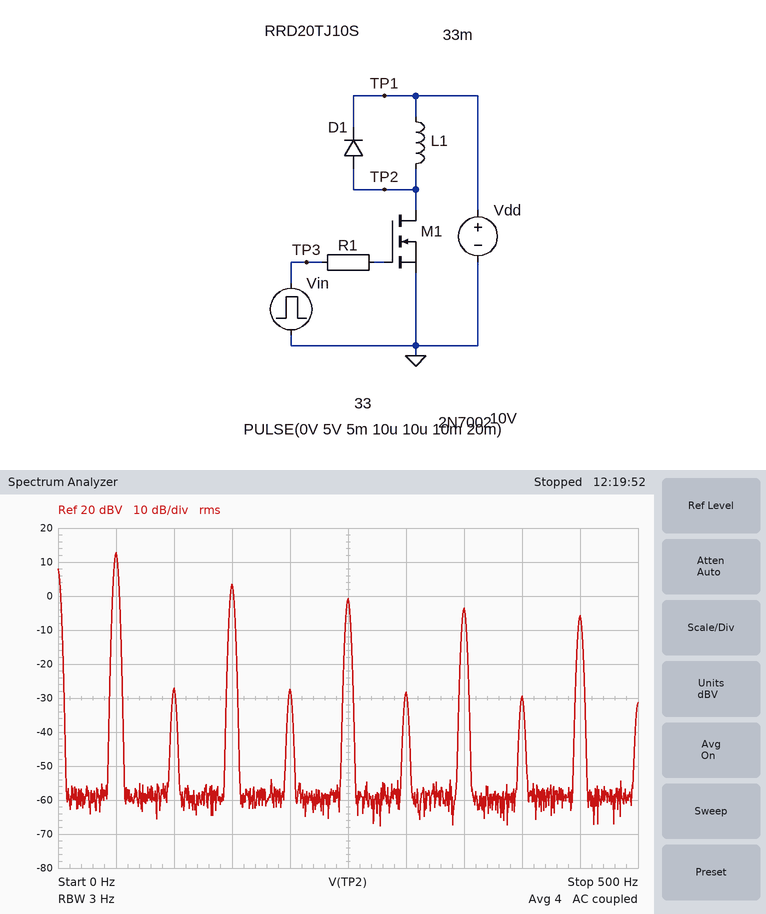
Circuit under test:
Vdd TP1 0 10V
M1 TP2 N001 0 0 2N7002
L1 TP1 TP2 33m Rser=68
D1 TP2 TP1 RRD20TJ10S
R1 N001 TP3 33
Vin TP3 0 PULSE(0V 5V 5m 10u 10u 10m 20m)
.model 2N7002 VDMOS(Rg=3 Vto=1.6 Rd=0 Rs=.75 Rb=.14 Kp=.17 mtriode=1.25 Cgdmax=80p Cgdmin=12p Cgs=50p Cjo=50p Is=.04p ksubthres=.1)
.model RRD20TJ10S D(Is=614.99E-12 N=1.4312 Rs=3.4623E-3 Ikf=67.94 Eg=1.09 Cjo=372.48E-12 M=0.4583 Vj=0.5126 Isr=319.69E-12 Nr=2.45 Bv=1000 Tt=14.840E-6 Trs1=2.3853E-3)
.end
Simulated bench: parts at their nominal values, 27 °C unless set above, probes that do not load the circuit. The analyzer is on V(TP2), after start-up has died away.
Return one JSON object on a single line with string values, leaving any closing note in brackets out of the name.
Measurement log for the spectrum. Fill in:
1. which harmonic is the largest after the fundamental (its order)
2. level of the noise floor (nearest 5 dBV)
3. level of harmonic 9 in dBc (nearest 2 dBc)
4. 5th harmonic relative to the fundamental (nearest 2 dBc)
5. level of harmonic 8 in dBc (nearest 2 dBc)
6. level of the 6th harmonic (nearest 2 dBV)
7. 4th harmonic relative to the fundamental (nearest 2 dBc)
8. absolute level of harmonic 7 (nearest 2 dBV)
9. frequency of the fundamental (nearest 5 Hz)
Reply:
{"which harmonic is the largest after the fundamental": "3", "level of the noise floor": "-60 dBV", "level of harmonic 9 in dBc": "-18 dBc", "5th harmonic relative to the fundamental": "-14 dBc", "level of harmonic 8 in dBc": "-42 dBc", "level of the 6th harmonic": "-28 dBV", "4th harmonic relative to the fundamental": "-40 dBc", "absolute level of harmonic 7": "-4 dBV", "frequency of the fundamental": "50 Hz"}
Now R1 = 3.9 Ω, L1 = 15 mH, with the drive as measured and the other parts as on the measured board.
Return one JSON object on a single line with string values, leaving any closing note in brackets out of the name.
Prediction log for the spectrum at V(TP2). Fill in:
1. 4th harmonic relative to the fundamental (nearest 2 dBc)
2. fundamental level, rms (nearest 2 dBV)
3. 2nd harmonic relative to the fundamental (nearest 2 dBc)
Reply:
{"4th harmonic relative to the fundamental": "-48 dBc", "fundamental level, rms": "12 dBV", "2nd harmonic relative to the fundamental": "-48 dBc"}
